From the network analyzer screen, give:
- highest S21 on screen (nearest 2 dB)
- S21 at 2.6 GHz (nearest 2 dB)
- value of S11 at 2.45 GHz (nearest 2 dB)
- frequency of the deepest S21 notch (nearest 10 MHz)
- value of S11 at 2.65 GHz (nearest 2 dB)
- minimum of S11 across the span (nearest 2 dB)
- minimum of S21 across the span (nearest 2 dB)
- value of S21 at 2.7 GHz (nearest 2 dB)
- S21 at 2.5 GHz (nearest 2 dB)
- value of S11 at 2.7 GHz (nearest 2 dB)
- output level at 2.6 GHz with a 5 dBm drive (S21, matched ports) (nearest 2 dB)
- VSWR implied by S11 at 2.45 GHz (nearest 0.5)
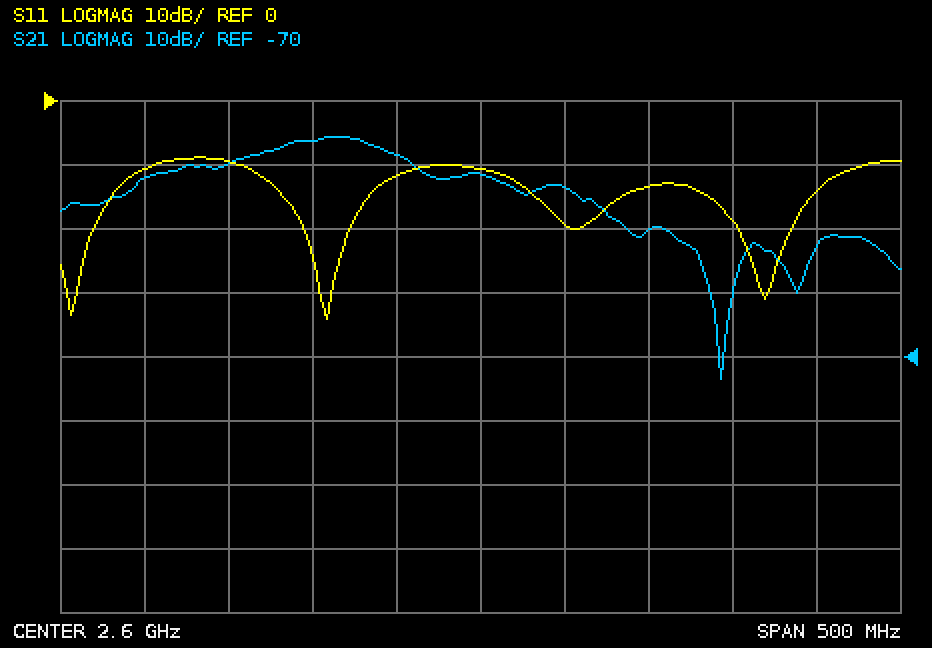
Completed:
-36 dB
-42 dB
-10 dB
2.74 GHz
-20 dB
-34 dB
-74 dB
-50 dB
-36 dB
-14 dB
-36 dBm
2.0
